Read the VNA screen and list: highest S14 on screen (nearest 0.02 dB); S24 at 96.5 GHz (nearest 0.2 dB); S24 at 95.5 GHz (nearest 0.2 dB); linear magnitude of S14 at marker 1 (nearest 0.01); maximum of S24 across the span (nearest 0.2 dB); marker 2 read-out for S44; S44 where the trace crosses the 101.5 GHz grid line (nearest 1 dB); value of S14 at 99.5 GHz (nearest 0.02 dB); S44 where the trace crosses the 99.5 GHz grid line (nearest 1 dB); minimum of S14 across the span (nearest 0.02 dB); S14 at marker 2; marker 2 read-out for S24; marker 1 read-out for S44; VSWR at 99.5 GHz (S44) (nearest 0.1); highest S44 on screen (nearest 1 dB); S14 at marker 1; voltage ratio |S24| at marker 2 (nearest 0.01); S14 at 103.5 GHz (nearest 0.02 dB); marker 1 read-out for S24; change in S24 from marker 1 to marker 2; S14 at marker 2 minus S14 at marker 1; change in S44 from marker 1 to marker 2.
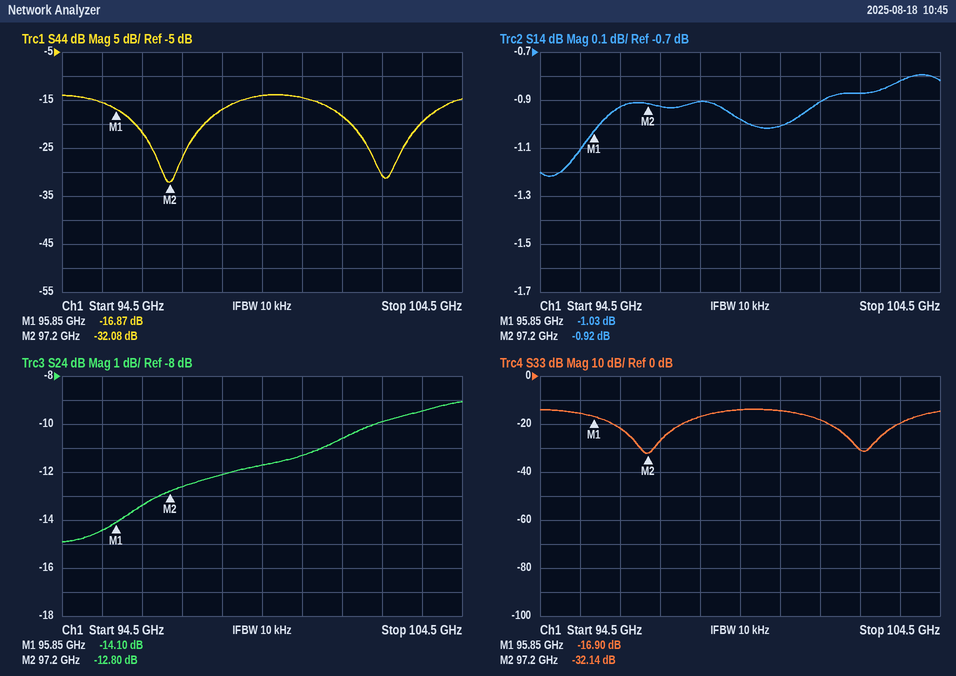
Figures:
-0.80 dB
-13.4 dB
-14.4 dB
0.89
-9.0 dB
-32.08 dB
-18 dB
-0.98 dB
-14 dB
-1.22 dB
-0.92 dB
-12.80 dB
-16.87 dB
1.5
-14 dB
-1.03 dB
0.23
-0.82 dB
-14.10 dB
1.30 dB
0.11 dB
-15.21 dB
